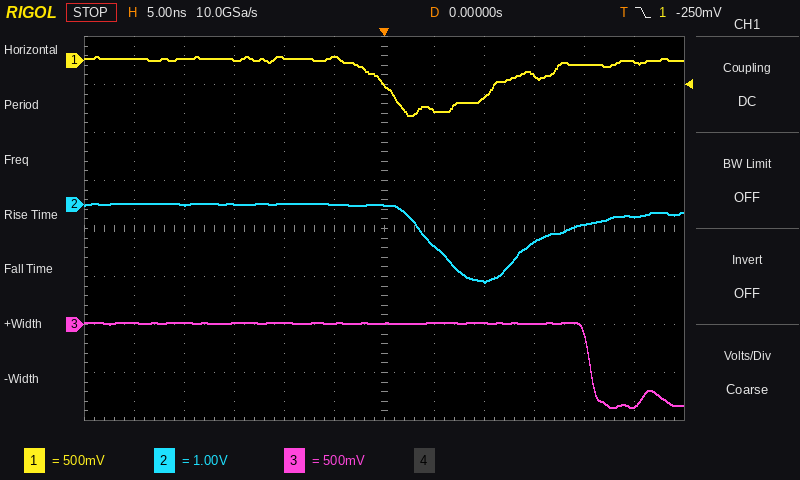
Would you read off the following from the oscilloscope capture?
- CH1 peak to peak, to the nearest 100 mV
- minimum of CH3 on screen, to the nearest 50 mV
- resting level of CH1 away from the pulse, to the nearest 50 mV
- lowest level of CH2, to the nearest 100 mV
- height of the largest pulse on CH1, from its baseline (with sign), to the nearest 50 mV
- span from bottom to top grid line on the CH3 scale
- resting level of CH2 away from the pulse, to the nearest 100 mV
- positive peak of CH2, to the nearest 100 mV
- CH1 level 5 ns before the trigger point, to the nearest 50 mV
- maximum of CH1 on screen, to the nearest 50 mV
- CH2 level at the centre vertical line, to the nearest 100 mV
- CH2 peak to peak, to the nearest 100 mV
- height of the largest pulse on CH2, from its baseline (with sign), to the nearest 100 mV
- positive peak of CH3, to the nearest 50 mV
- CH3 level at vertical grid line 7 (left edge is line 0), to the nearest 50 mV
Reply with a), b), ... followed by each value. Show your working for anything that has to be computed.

a) 600 mV
b) -850 mV
c) 0 mV
d) -1.6 V
e) -600 mV
f) 4 V
g) 0.0 V
h) 0.0 V
i) 50 mV
j) 50 mV
k) 0.0 V
l) 0.0 V − (-1.6 V) = 1.6 V
m) -1.6 V − (0.0 V) = -1.6 V
n) 0 mV
o) 0 mV
